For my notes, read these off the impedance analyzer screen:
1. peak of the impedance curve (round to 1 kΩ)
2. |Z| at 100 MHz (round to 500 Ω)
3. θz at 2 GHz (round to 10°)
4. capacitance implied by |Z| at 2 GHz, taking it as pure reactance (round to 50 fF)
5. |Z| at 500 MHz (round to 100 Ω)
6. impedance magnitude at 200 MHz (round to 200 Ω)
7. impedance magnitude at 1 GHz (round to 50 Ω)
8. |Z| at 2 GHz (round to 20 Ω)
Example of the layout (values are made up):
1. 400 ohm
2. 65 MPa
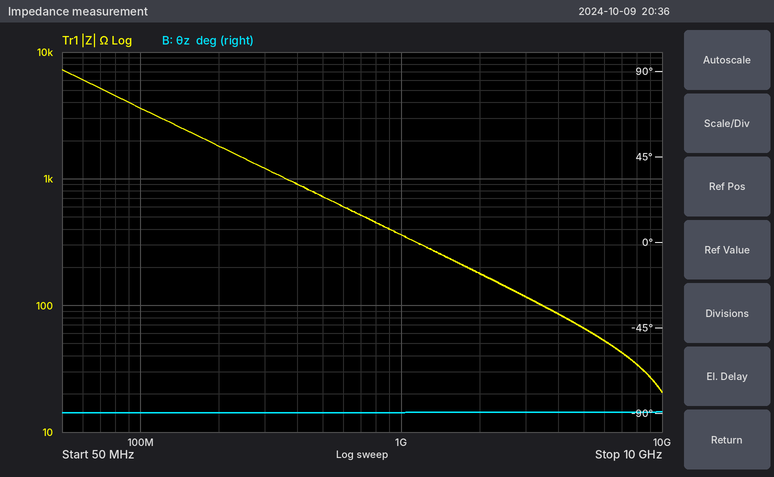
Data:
1. 7 kΩ
2. 3.5 kΩ
3. -90°
4. 450 fF
5. 700 Ω
6. 1.8 kΩ
7. 350 Ω
8. 180 Ω
